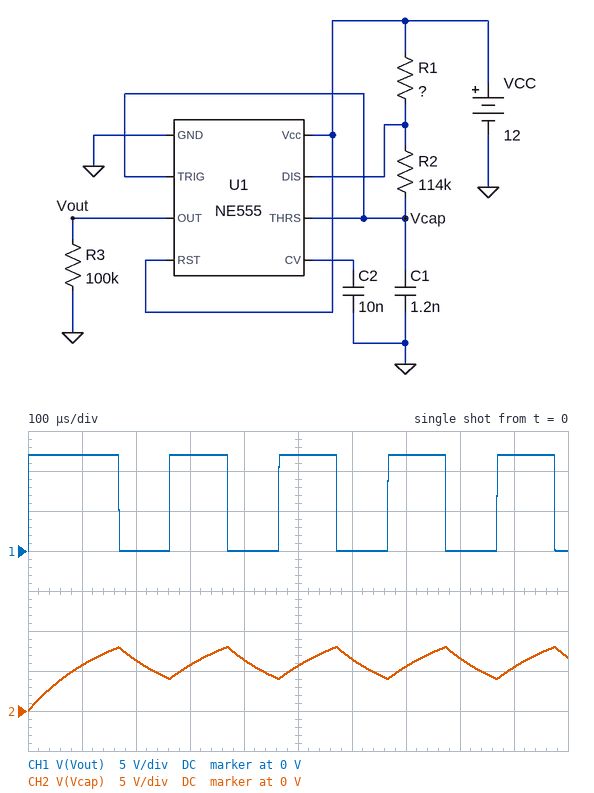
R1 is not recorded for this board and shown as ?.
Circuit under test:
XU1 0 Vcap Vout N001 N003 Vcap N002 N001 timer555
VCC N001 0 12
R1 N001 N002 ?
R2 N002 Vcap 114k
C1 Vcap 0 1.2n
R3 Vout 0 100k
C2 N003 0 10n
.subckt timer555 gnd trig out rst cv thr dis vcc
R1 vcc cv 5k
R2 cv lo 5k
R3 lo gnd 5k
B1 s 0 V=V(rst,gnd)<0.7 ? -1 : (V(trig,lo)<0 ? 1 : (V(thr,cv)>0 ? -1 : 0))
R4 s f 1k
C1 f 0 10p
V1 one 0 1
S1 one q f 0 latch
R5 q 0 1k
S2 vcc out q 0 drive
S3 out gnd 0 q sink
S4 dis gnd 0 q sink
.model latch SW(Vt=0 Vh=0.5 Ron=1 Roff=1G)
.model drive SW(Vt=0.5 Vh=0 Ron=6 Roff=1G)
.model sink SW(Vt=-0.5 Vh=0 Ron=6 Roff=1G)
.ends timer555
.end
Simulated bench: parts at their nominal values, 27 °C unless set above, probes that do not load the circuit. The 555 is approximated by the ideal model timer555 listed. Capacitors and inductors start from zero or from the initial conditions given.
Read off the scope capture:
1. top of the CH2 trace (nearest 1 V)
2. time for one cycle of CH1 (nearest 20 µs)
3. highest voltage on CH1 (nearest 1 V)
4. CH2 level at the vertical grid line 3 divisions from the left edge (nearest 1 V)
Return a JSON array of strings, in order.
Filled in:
["8 V", "200 µs", "12 V", "6 V"]
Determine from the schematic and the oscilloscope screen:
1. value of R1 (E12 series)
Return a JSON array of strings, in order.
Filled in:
["15 kΩ"]
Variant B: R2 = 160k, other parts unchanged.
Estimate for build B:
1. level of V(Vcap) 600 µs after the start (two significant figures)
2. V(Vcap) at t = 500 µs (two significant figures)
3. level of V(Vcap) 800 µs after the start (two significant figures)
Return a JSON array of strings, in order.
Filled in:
["5.0 V", "7.8 V", "7.5 V"]
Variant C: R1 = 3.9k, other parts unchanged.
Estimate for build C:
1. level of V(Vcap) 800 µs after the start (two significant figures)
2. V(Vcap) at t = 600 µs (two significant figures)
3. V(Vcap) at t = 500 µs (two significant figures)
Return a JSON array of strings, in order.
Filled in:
["4.8 V", "5.1 V", "6.8 V"]
